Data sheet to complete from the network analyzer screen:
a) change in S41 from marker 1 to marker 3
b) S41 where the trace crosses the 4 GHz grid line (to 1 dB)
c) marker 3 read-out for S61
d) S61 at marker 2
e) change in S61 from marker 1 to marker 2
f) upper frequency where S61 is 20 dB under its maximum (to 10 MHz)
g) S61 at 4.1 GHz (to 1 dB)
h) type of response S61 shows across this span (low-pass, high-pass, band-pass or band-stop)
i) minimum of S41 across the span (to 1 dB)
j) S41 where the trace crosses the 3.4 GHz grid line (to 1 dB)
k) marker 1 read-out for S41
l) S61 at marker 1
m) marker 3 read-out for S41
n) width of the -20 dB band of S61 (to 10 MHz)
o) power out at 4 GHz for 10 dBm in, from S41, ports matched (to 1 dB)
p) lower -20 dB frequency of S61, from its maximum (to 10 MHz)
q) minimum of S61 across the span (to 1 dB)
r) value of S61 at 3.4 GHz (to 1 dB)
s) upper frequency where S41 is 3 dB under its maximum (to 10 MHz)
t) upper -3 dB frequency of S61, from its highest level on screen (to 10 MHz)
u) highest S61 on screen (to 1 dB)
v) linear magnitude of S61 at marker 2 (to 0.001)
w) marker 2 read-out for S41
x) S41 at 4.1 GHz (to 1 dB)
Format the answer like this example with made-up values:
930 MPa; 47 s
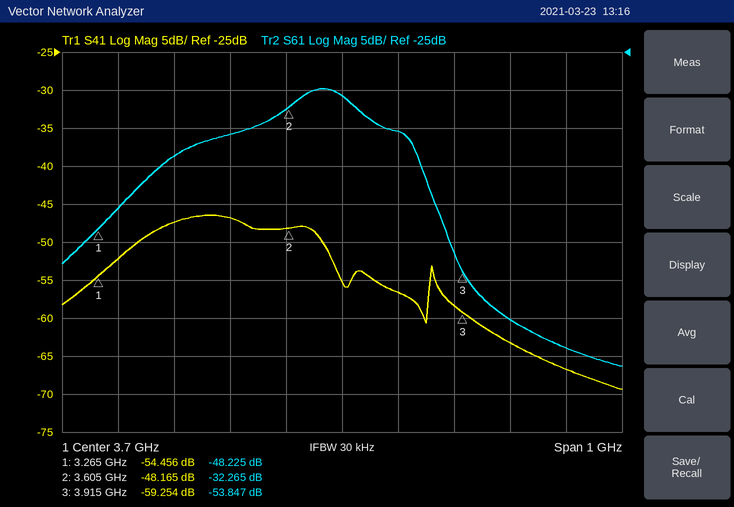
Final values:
-4.798 dB; -63 dB; -53.847 dB; -32.265 dB; 15.960 dB; 3.89 GHz; -64 dB; band-pass; -69 dB; -47 dB; -54.456 dB; -48.225 dB; -59.254 dB; 650 MHz; -53 dBm; 3.24 GHz; -66 dB; -39 dB; 3.66 GHz; 3.73 GHz; -30 dB; 0.024; -48.165 dB; -67 dB
